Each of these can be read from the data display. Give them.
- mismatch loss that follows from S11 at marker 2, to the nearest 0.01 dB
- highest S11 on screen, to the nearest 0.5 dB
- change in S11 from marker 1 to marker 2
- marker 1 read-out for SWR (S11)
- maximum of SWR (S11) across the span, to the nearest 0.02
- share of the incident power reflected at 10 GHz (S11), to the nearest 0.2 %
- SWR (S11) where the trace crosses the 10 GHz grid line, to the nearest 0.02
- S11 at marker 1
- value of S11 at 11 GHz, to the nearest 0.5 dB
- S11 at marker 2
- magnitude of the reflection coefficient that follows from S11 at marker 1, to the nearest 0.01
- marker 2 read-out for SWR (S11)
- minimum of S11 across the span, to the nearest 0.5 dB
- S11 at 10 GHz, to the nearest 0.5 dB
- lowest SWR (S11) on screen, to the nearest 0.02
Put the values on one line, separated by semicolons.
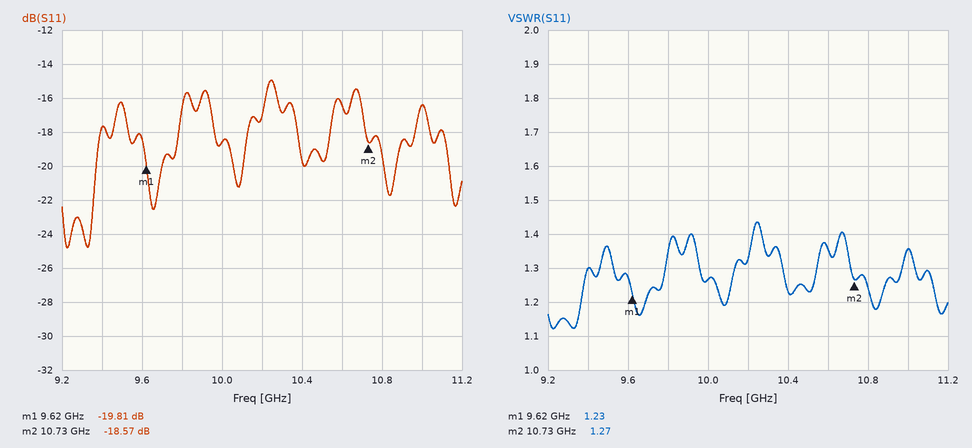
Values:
0.06 dB; -15.0 dB; 1.24 dB; 1.23; 1.44; 1.4 %; 1.26; -19.81 dB; -16.5 dB; -18.57 dB; 0.10; 1.27; -25.0 dB; -18.5 dB; 1.12
